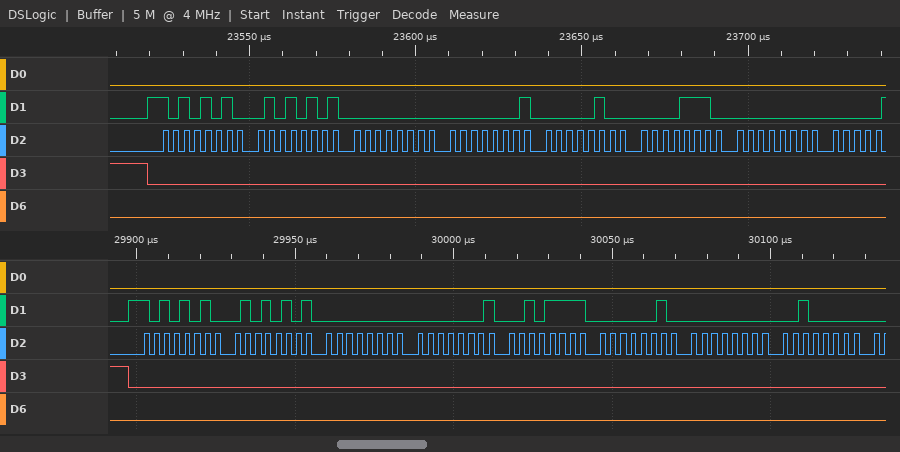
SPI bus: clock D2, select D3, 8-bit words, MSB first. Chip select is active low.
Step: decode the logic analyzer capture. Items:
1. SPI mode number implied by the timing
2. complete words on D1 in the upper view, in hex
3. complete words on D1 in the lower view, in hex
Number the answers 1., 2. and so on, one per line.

1. 0
2. AA, 55, 00, 01, 04, 0E, 00
3. AA, 55, 00, 01, 2F, 02, 00, 20
